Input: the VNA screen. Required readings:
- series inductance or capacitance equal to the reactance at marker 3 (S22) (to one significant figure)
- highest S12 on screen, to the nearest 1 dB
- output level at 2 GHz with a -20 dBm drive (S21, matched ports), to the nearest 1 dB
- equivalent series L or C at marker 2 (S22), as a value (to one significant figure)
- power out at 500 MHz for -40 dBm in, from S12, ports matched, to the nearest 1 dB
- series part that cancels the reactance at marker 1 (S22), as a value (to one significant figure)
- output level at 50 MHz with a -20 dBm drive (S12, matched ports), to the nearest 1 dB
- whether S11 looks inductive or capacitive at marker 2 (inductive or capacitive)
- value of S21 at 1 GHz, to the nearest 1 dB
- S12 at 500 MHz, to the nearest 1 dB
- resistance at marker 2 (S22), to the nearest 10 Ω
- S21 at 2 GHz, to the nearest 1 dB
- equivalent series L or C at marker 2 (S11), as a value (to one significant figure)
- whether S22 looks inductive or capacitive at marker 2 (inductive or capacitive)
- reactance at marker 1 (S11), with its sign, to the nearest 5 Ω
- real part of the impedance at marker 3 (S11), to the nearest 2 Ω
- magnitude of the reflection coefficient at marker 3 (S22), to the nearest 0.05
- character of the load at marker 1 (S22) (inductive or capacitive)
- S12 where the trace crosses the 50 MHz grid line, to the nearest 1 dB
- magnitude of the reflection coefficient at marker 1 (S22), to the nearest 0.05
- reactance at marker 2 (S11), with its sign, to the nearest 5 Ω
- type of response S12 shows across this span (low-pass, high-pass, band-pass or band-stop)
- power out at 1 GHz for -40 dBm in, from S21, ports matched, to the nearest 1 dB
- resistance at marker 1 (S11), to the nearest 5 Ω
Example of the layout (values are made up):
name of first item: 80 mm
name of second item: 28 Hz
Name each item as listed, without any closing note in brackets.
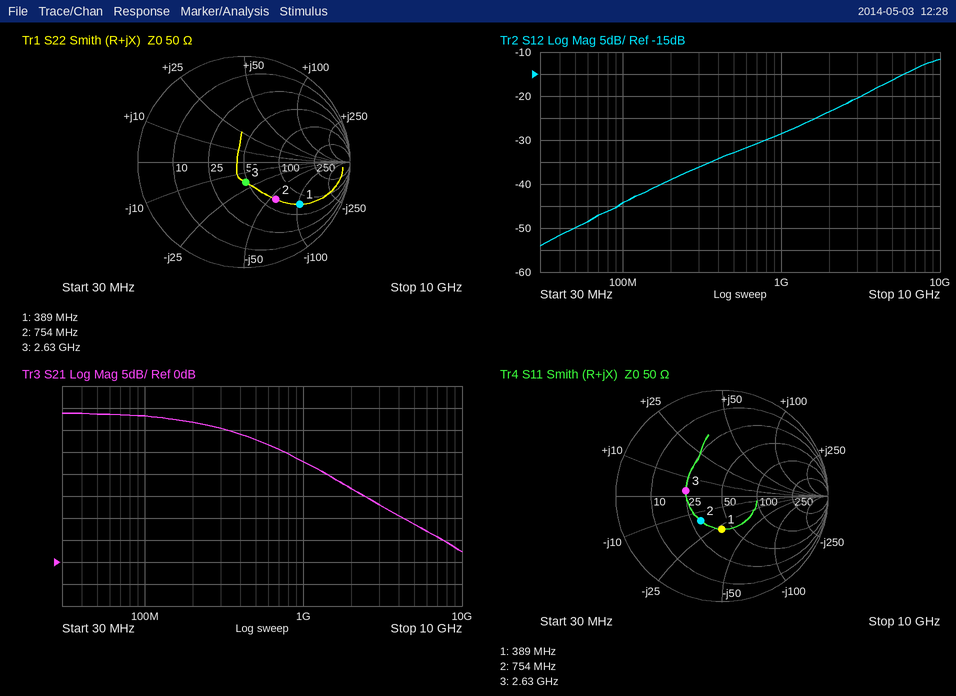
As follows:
series inductance or capacitance equal to the reactance at marker 3 (S22): 3 pF
highest S12 on screen, to the nearest 1 dB: -12 dB
output level at 2 GHz with a -20 dBm drive (S21, matched ports), to the nearest 1 dB: -3 dBm
equivalent series L or C at marker 2 (S22), as a value: 4 pF
power out at 500 MHz for -40 dBm in, from S12, ports matched, to the nearest 1 dB: -73 dBm
series part that cancels the reactance at marker 1 (S22), as a value: 40 nH
output level at 50 MHz with a -20 dBm drive (S12, matched ports), to the nearest 1 dB: -70 dBm
whether S11 looks inductive or capacitive at marker 2: capacitive
value of S21 at 1 GHz, to the nearest 1 dB: 23 dB
S12 at 500 MHz, to the nearest 1 dB: -33 dB
resistance at marker 2 (S22), to the nearest 10 Ω: 60 Ω
S21 at 2 GHz, to the nearest 1 dB: 17 dB
equivalent series L or C at marker 2 (S11), as a value: 10 pF
whether S22 looks inductive or capacitive at marker 2: capacitive
reactance at marker 1 (S11), with its sign, to the nearest 5 Ω: -30 Ω
real part of the impedance at marker 3 (S11), to the nearest 2 Ω: 24 Ω
magnitude of the reflection coefficient at marker 3 (S22), to the nearest 0.05: 0.20
character of the load at marker 1 (S22): capacitive
S12 where the trace crosses the 50 MHz grid line, to the nearest 1 dB: -50 dB
magnitude of the reflection coefficient at marker 1 (S22), to the nearest 0.05: 0.65
reactance at marker 2 (S11), with its sign, to the nearest 5 Ω: -15 Ω
type of response S12 shows across this span: high-pass
power out at 1 GHz for -40 dBm in, from S21, ports matched, to the nearest 1 dB: -17 dBm
resistance at marker 1 (S11), to the nearest 5 Ω: 40 Ω
